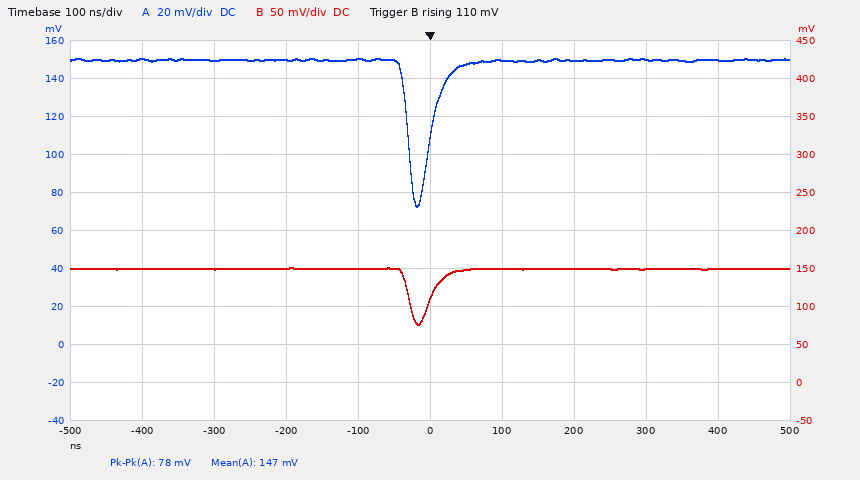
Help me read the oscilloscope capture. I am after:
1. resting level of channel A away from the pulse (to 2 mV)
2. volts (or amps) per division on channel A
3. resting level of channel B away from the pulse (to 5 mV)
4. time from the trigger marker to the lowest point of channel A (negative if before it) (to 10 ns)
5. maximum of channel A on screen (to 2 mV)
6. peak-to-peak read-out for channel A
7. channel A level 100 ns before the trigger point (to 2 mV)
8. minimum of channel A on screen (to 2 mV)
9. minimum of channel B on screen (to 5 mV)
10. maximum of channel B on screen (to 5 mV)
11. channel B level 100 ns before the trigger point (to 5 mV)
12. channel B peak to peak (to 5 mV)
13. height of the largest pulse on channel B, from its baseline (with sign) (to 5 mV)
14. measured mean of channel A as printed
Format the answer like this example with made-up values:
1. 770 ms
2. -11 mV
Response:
1. 150 mV
2. 20 mV
3. 150 mV
4. -20 ns
5. 150 mV
6. 78 mV
7. 150 mV
8. 72 mV
9. 75 mV
10. 150 mV
11. 150 mV
12. 75 mV
13. -75 mV
14. 147 mV
